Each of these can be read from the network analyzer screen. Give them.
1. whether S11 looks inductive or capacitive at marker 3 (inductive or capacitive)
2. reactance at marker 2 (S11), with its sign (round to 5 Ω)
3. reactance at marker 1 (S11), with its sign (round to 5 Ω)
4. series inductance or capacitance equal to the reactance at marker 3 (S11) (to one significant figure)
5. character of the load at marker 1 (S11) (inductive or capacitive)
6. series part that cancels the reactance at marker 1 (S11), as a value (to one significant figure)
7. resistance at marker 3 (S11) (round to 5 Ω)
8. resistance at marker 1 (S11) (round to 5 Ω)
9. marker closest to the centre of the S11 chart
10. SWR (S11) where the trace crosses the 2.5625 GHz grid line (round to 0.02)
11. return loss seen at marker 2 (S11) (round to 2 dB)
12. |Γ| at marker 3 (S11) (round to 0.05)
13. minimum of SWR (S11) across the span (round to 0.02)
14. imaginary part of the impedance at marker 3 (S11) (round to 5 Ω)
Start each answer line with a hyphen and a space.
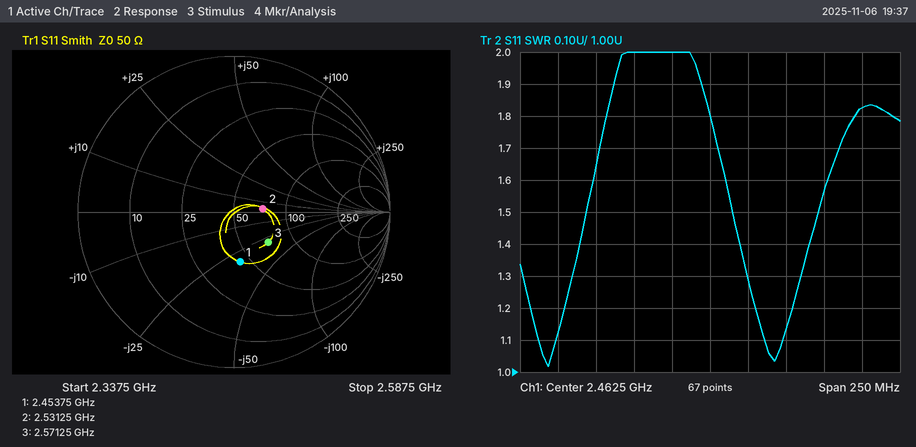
- capacitive
- +5 Ω
- -30 Ω
- 2 pF
- capacitive
- 2 nH
- 70 Ω
- 45 Ω
- marker 2
- 1.82
- 14 dB
- 0.30
- 1.02
- -30 Ω
